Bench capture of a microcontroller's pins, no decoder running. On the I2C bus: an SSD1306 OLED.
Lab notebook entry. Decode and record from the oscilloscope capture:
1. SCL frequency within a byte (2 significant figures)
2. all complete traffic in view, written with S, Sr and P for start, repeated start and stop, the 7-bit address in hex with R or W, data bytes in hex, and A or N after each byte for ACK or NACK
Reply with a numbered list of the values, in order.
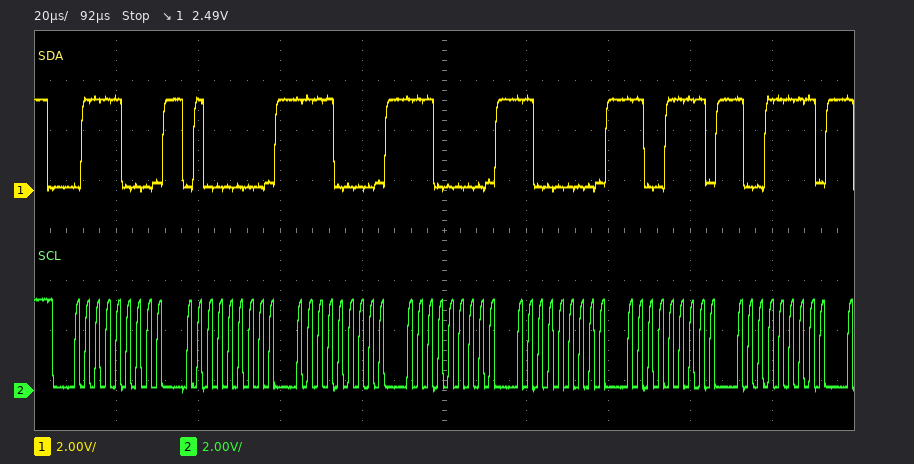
1. 400 kHz
2. S 3CW A 40 A F0 A E0 A C0 A CF A 9F A
